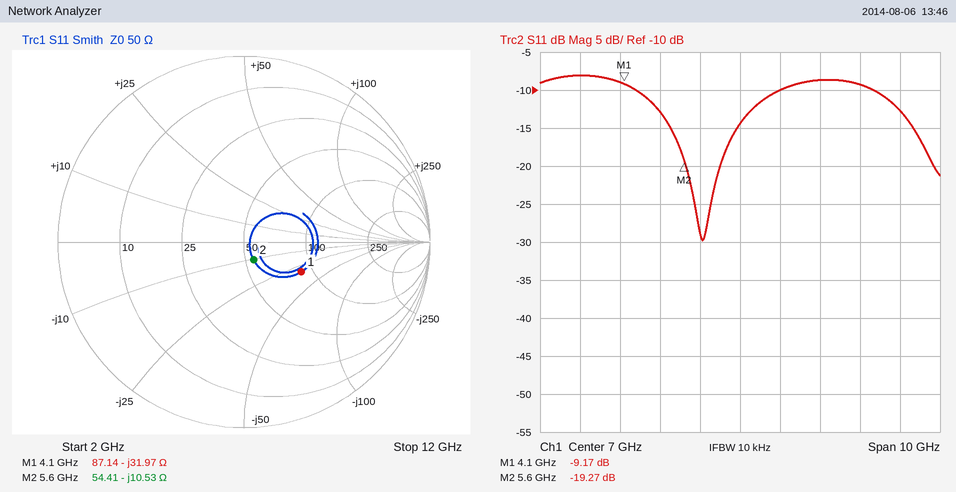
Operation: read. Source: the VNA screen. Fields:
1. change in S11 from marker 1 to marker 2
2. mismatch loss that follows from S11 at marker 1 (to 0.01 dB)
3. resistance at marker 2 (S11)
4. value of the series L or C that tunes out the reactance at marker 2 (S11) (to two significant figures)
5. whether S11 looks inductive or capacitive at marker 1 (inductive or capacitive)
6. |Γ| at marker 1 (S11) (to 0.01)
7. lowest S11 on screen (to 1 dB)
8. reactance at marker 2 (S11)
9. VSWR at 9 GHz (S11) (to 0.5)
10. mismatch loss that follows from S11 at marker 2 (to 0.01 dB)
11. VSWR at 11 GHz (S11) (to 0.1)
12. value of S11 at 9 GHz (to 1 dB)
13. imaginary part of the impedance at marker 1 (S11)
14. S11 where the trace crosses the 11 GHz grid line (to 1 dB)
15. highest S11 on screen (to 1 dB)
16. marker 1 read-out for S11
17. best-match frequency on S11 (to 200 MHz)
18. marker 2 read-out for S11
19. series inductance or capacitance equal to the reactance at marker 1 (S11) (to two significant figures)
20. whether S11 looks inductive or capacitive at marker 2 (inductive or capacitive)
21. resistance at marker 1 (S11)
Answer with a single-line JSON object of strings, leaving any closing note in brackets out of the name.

{"change in S11 from marker 1 to marker 2": "-10.10 dB", "mismatch loss that follows from S11 at marker 1": "0.56 dB", "resistance at marker 2": "54.41 Ω", "value of the series L or C that tunes out the reactance at marker 2 (S11)": "300 pH", "whether S11 looks inductive or capacitive at marker 1": "capacitive", "|Γ| at marker 1 (S11)": "0.35", "lowest S11 on screen": "-30 dB", "reactance at marker 2": "-10.53 Ω", "VSWR at 9 GHz (S11)": "2.0", "mismatch loss that follows from S11 at marker 2": "0.05 dB", "VSWR at 11 GHz (S11)": "1.6", "value of S11 at 9 GHz": "-9 dB", "imaginary part of the impedance at marker 1": "-31.97 Ω", "S11 where the trace crosses the 11 GHz grid line": "-13 dB", "highest S11 on screen": "-8 dB", "marker 1 read-out for S11": "-9.17 dB", "best-match frequency on S11": "6.0 GHz", "marker 2 read-out for S11": "-19.27 dB", "series inductance or capacitance equal to the reactance at marker 1 (S11)": "1.2 pF", "whether S11 looks inductive or capacitive at marker 2": "capacitive", "resistance at marker 1": "87.14 Ω"}
